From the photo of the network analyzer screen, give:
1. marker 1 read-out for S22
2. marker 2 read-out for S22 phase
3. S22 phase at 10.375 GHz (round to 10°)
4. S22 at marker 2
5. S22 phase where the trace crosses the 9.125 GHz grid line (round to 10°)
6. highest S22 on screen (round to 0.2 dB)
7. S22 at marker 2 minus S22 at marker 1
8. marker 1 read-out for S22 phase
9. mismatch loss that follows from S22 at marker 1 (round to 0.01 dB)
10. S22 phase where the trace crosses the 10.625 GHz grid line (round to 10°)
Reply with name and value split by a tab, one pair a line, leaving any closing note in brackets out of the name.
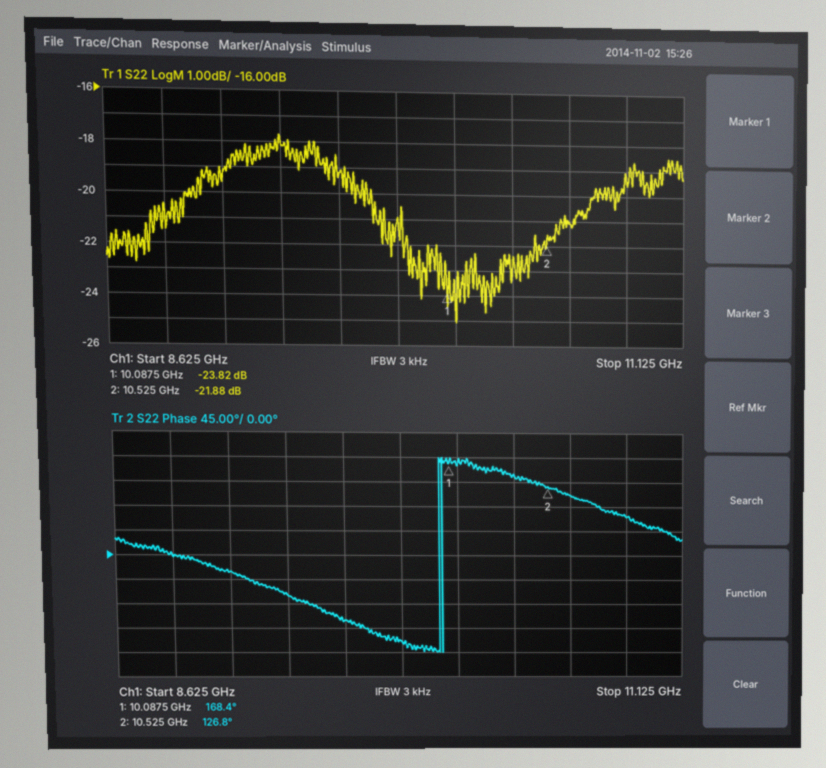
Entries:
marker 1 read-out for S22	-23.82 dB
marker 2 read-out for S22 phase	126.8°
S22 phase at 10.375 GHz	150°
S22 at marker 2	-21.88 dB
S22 phase where the trace crosses the 9.125 GHz grid line	-30°
highest S22 on screen	-17.8 dB
S22 at marker 2 minus S22 at marker 1	1.94 dB
marker 1 read-out for S22 phase	168.4°
mismatch loss that follows from S22 at marker 1	0.02 dB
S22 phase where the trace crosses the 10.625 GHz grid line	110°
